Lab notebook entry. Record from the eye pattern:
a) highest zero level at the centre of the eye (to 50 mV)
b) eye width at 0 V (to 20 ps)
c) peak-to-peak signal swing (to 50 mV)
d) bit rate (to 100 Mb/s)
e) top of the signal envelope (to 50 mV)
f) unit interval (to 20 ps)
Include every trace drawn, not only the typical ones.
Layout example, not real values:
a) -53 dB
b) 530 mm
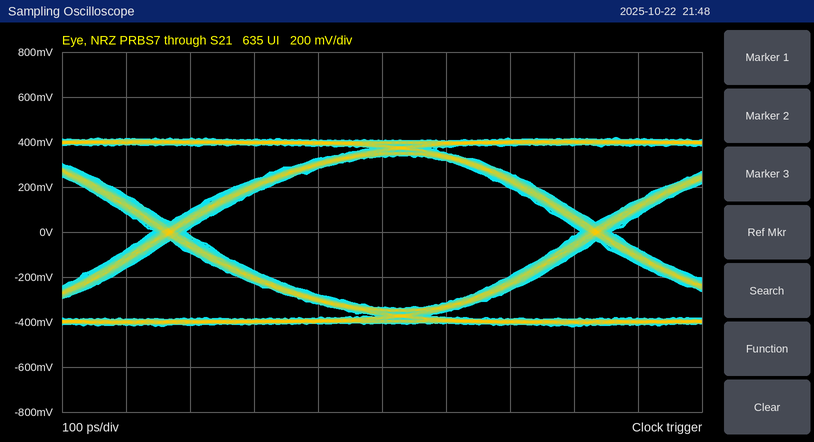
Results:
a) -350 mV
b) 620 ps
c) 850 mV
d) 1.5 Gb/s
e) 400 mV
f) 660 ps
